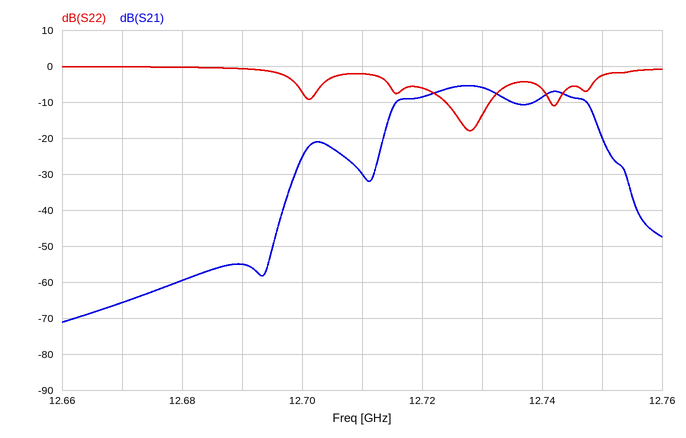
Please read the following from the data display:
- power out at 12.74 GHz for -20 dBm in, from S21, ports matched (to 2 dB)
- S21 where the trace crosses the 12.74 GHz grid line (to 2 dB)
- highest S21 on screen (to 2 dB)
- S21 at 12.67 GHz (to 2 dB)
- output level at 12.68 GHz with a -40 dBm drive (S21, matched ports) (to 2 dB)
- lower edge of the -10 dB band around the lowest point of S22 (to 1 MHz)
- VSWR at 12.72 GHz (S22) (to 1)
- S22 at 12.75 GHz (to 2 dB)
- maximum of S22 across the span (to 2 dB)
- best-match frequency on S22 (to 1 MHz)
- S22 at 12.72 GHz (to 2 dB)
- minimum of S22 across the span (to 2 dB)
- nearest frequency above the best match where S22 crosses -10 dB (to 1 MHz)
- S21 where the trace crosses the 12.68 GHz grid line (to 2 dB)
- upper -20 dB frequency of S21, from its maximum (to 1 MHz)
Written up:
-28 dBm
-8 dB
-6 dB
-66 dB
-100 dBm
12.724 GHz
3
-2 dB
0 dB
12.728 GHz
-6 dB
-18 dB
12.731 GHz
-60 dB
12.752 GHz
